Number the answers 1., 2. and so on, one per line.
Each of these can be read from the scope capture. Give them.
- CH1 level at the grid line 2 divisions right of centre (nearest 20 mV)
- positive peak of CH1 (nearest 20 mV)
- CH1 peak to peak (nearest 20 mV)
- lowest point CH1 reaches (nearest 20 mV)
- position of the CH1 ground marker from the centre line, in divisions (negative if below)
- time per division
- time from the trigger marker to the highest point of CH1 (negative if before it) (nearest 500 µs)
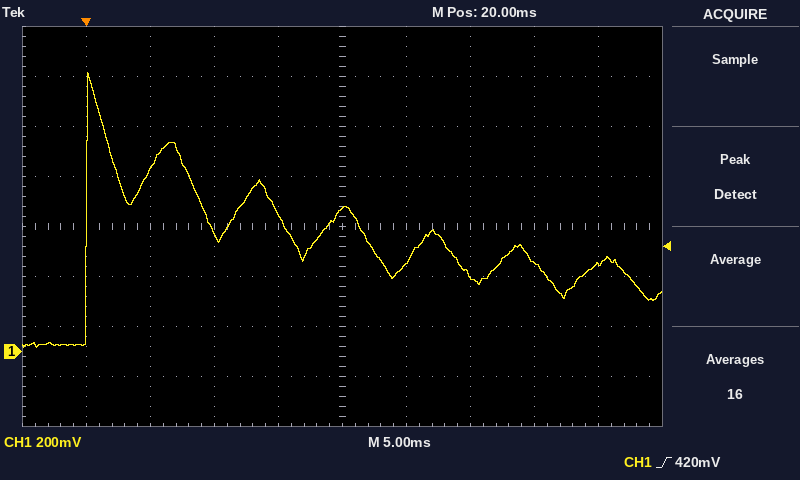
1. 300 mV
2. 1.12 V
3. 1.10 V
4. 20 mV
5. -2.5 div
6. 5 ms
7. 0.0 ms
